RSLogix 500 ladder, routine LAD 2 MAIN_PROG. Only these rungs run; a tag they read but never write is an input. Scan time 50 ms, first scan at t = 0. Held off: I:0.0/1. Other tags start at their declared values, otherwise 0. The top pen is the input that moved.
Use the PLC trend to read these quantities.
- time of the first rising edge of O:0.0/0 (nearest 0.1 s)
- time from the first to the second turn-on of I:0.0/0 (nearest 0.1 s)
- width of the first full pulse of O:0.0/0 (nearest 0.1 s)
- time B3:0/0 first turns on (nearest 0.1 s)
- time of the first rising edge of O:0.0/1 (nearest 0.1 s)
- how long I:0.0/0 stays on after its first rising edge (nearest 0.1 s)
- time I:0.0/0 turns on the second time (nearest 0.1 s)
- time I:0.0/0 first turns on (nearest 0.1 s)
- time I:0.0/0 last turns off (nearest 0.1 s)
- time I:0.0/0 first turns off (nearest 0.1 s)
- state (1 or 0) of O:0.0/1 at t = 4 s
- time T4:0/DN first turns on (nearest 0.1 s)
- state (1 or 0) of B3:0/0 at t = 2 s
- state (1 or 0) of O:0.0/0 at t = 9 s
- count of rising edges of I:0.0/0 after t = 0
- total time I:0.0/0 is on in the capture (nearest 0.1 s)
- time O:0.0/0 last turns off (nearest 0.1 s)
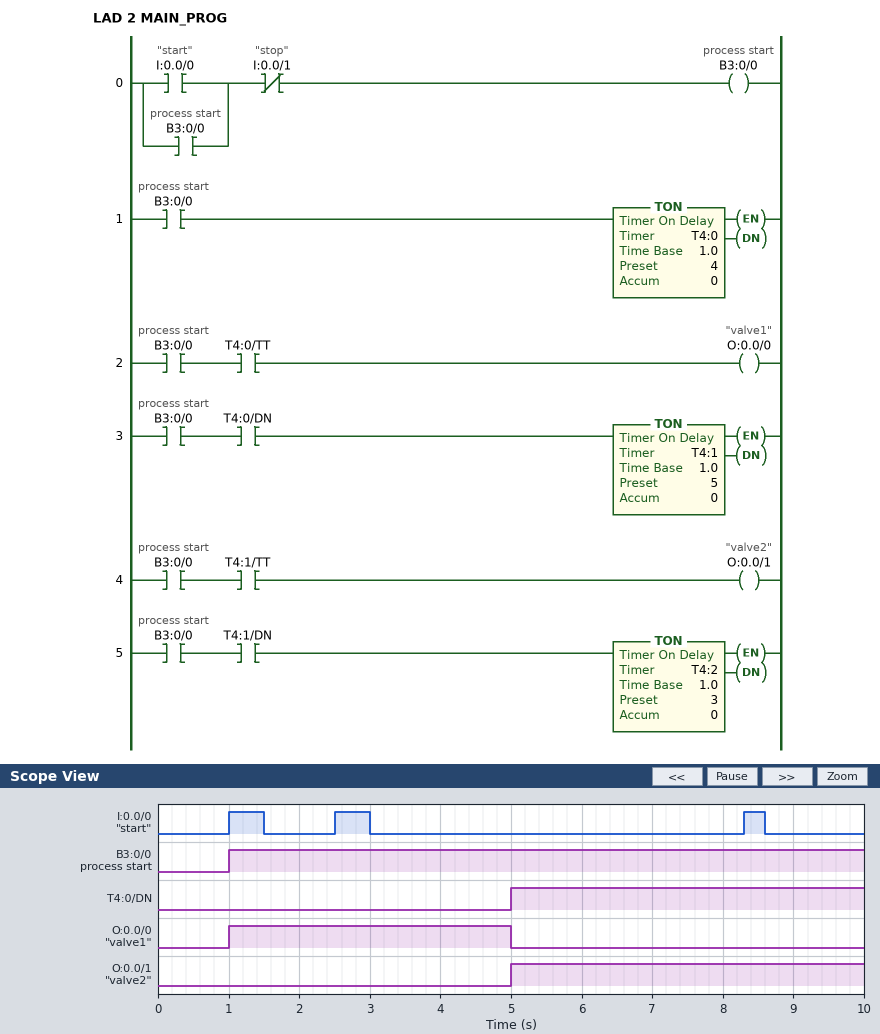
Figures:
1.0 s
1.5 s
4.0 s
1.0 s
5.0 s
0.5 s
2.5 s
1.0 s
8.6 s
1.5 s
0
5.0 s
1
0
3
1.3 s
5.0 s
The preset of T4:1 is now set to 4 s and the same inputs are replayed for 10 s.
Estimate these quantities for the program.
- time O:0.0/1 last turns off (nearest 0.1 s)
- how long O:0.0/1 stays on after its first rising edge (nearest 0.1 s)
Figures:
9.0 s
4.0 s
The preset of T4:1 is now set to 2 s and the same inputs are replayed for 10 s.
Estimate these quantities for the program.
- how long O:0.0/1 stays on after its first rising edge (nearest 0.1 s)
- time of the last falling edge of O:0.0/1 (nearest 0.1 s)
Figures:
2.0 s
7.0 s
